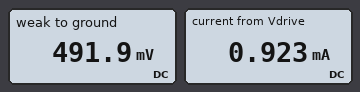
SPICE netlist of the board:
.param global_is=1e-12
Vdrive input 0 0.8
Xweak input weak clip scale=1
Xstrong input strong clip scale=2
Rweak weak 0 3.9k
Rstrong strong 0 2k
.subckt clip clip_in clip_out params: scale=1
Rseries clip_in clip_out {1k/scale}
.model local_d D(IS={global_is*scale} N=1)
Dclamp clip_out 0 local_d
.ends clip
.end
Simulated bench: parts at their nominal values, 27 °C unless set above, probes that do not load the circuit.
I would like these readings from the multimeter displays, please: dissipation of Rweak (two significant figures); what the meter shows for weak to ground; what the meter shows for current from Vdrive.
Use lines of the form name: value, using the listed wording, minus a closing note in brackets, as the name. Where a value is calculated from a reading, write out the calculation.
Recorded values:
dissipation of Rweak: (491.9 mV)^2 / 3.9 kΩ = 62 µW
what the meter shows for weak to ground: 491.9 mV
what the meter shows for current from Vdrive: 0.923 mA
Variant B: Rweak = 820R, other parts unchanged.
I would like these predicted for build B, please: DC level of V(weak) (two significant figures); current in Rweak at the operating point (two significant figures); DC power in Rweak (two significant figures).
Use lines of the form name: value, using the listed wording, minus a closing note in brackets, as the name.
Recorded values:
DC level of V(weak): 360 mV
current in Rweak at the operating point: 440 µA
DC power in Rweak: 160 µW
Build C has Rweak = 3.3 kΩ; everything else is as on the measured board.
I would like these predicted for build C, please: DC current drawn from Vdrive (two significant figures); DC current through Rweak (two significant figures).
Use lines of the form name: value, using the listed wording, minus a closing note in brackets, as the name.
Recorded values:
DC current drawn from Vdrive: 930 µA
DC current through Rweak: 150 µA
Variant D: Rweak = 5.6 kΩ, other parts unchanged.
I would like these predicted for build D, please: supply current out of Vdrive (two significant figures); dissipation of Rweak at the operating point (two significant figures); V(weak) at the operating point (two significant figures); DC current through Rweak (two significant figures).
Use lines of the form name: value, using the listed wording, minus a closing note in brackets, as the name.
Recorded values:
supply current out of Vdrive: 920 µA
dissipation of Rweak at the operating point: 44 µW
V(weak) at the operating point: 500 mV
DC current through Rweak: 89 µA
